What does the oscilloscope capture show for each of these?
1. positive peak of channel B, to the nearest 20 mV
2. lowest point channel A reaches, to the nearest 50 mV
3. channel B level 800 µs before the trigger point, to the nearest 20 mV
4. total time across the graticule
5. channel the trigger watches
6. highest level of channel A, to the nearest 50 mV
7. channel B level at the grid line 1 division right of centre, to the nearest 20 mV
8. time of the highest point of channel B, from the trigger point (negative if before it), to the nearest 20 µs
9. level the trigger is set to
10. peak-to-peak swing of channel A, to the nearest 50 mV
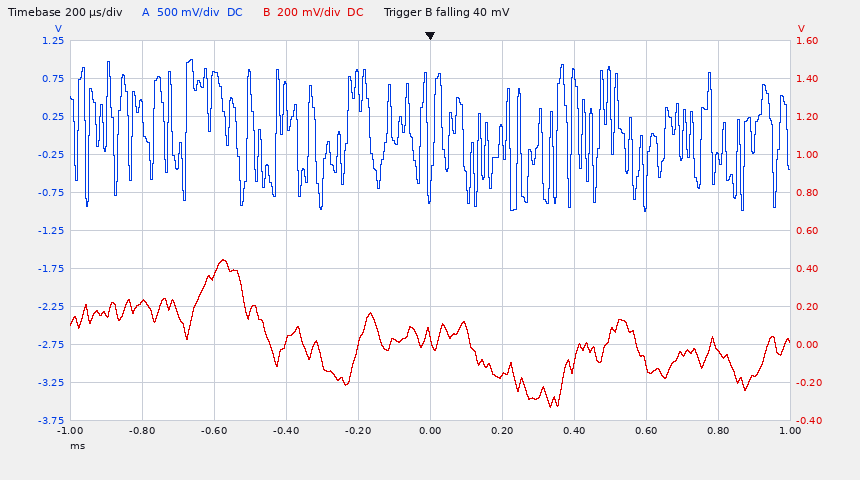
440 mV
-1.00 V
220 mV
2 ms
channel B
1.00 V
-160 mV
-580 µs
40 mV
2.00 V
